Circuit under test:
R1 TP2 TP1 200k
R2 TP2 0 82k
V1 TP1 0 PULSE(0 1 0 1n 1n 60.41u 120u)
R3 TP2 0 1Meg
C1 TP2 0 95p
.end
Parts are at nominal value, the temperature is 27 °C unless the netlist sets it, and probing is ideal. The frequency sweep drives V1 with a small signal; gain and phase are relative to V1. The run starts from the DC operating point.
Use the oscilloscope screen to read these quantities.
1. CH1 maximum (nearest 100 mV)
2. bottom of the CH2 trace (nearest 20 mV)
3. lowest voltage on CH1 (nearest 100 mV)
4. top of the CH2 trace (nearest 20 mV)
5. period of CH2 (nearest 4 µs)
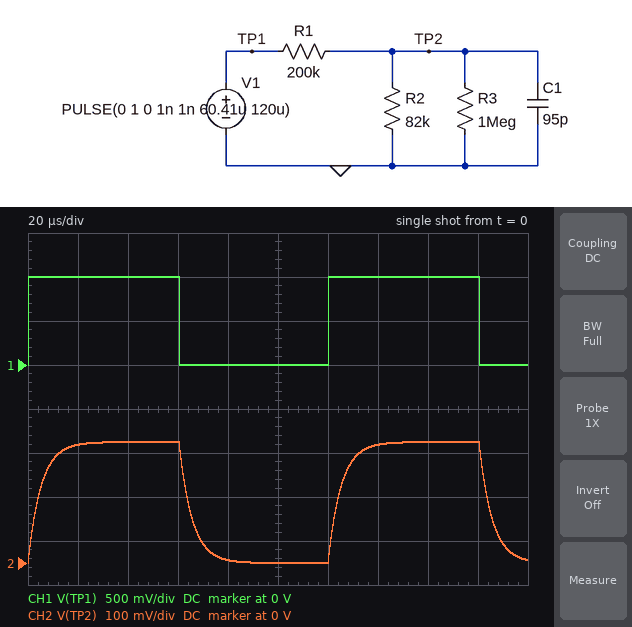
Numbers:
1.0 V
0 V
0 V
280 mV
120 µs
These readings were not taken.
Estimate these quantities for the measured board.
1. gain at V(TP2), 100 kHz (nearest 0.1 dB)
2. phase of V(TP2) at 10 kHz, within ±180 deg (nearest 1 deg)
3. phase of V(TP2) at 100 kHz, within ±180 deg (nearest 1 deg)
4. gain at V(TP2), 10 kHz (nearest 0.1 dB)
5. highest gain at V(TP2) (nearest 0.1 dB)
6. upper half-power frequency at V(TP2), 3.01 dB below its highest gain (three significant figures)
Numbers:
-21.9 dB
-18 deg
-73 deg
-11.7 dB
-11.2 dB
30.5 kHz
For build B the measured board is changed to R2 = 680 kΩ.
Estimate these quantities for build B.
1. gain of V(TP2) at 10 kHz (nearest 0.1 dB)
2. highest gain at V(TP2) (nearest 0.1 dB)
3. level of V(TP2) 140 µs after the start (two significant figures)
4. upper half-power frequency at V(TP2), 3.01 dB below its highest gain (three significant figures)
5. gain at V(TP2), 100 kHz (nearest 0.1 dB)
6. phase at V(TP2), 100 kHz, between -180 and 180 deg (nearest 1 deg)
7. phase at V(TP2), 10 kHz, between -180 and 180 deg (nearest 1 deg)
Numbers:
-5.6 dB
-3.5 dB
530 mV
12.5 kHz
-21.6 dB
-83 deg
-39 deg
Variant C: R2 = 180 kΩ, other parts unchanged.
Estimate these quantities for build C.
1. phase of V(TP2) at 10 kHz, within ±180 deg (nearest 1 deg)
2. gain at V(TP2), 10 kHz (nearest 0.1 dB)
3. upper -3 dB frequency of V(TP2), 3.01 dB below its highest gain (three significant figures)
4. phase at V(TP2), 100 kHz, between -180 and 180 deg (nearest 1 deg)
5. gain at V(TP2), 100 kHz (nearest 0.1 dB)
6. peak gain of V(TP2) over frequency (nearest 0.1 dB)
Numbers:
-27 deg
-8.3 dB
19.4 kHz
-79 deg
-21.7 dB
-7.3 dB
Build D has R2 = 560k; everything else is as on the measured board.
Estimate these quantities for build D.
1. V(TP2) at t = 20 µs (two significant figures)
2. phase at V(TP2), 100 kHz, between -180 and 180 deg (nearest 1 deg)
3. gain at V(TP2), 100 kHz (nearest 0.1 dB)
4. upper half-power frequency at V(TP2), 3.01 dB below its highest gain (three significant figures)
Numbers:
520 mV
-83 deg
-21.6 dB
13.0 kHz
